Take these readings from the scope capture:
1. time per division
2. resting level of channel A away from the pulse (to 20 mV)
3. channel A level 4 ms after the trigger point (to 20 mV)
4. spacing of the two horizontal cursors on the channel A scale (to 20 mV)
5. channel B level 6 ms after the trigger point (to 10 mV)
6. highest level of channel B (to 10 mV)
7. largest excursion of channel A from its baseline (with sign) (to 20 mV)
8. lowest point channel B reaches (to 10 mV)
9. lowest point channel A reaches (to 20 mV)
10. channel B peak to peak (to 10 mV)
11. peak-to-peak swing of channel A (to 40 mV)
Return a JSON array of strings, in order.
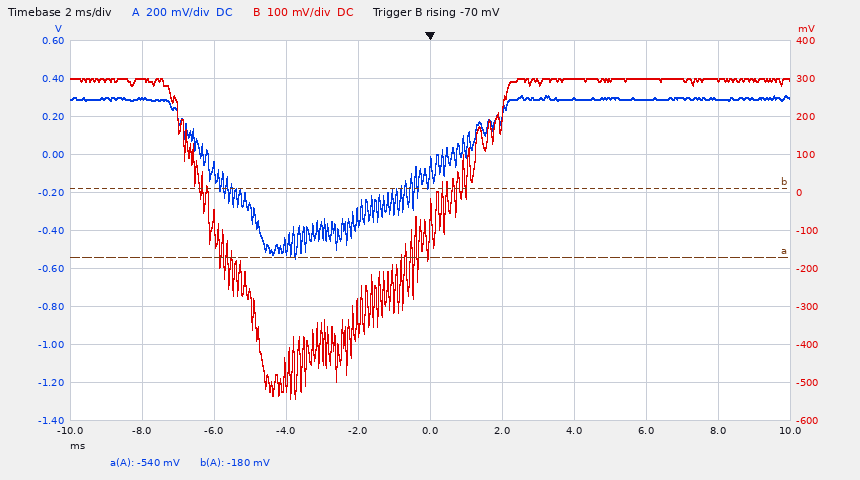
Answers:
["2 ms", "300 mV", "300 mV", "360 mV", "300 mV", "300 mV", "-840 mV", "-540 mV", "-540 mV", "840 mV", "840 mV"]
